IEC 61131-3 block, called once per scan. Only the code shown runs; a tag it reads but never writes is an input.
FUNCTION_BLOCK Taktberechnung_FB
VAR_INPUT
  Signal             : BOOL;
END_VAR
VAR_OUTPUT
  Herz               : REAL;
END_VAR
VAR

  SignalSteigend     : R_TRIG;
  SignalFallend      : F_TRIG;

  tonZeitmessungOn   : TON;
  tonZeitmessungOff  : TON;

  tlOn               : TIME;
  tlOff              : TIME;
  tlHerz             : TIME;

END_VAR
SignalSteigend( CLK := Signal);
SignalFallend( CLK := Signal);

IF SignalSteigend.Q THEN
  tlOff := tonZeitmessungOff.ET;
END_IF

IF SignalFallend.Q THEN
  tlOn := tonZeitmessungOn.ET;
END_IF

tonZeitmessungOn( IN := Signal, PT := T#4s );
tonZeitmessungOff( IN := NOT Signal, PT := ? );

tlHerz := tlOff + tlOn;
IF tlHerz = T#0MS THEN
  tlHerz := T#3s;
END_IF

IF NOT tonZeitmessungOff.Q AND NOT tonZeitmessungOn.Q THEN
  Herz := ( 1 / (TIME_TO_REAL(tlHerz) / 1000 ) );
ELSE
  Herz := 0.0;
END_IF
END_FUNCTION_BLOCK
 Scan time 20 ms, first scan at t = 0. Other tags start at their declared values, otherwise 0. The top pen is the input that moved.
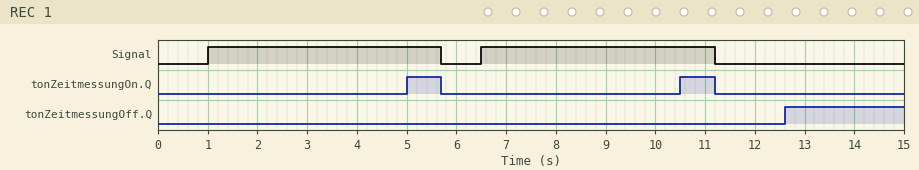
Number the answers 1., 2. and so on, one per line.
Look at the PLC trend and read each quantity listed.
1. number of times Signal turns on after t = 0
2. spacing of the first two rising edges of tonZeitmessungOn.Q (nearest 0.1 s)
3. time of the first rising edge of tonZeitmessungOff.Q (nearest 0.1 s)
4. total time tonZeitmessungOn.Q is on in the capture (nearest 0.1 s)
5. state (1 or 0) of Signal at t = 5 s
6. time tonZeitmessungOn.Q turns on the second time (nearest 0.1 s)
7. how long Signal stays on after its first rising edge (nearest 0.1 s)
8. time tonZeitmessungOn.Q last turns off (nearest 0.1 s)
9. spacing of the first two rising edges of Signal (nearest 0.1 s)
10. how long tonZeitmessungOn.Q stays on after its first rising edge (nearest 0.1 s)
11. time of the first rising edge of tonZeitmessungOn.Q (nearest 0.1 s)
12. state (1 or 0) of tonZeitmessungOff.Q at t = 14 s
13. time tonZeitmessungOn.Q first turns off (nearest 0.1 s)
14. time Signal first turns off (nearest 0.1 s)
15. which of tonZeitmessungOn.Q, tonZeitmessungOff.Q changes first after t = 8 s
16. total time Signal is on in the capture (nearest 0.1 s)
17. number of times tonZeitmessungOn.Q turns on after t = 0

1. 2
2. 5.5 s
3. 12.6 s
4. 1.4 s
5. 1
6. 10.5 s
7. 4.7 s
8. 11.2 s
9. 5.5 s
10. 0.7 s
11. 5.0 s
12. 1
13. 5.7 s
14. 5.7 s
15. tonZeitmessungOn.Q
16. 9.4 s
17. 2
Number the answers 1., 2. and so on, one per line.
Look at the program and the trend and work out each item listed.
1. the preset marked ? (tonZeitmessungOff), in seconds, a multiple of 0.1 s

1. 1.4 s
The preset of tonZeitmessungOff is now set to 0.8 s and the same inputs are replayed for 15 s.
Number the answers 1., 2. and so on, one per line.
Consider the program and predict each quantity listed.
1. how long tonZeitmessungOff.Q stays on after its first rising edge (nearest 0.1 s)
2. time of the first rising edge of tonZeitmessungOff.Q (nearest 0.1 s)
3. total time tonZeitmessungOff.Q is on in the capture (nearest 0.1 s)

1. 0.2 s
2. 0.8 s
3. 3.2 s
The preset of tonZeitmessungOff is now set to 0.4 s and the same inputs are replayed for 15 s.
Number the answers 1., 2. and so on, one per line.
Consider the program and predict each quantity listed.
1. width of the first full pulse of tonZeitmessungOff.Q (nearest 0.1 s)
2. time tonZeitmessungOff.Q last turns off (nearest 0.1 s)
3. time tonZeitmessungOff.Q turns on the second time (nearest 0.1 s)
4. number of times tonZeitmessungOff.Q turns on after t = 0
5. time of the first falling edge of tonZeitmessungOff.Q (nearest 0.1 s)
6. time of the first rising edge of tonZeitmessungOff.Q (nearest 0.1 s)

1. 0.6 s
2. 6.5 s
3. 6.1 s
4. 3
5. 1.0 s
6. 0.4 s
